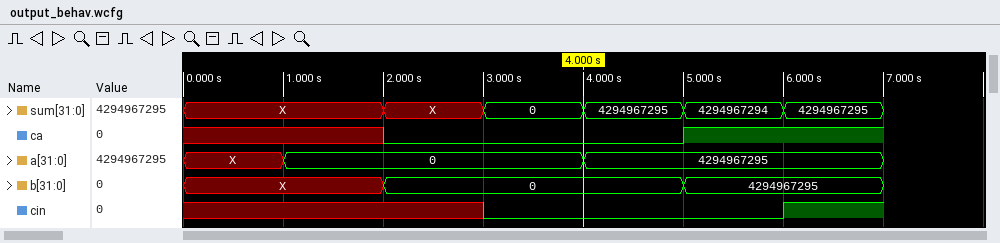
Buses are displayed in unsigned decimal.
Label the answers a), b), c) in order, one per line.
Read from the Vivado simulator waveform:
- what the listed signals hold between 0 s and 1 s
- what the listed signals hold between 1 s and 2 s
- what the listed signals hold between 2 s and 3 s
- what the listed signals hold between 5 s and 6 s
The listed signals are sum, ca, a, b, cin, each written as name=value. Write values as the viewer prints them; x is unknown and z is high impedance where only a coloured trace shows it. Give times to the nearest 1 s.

a) sum=X, ca=x, a=X, b=X, cin=x
b) sum=X, ca=x, a=0, b=X, cin=x
c) sum=X, ca=0, a=0, b=0, cin=x
d) sum=4294967294, ca=1, a=4294967295, b=4294967295, cin=0
